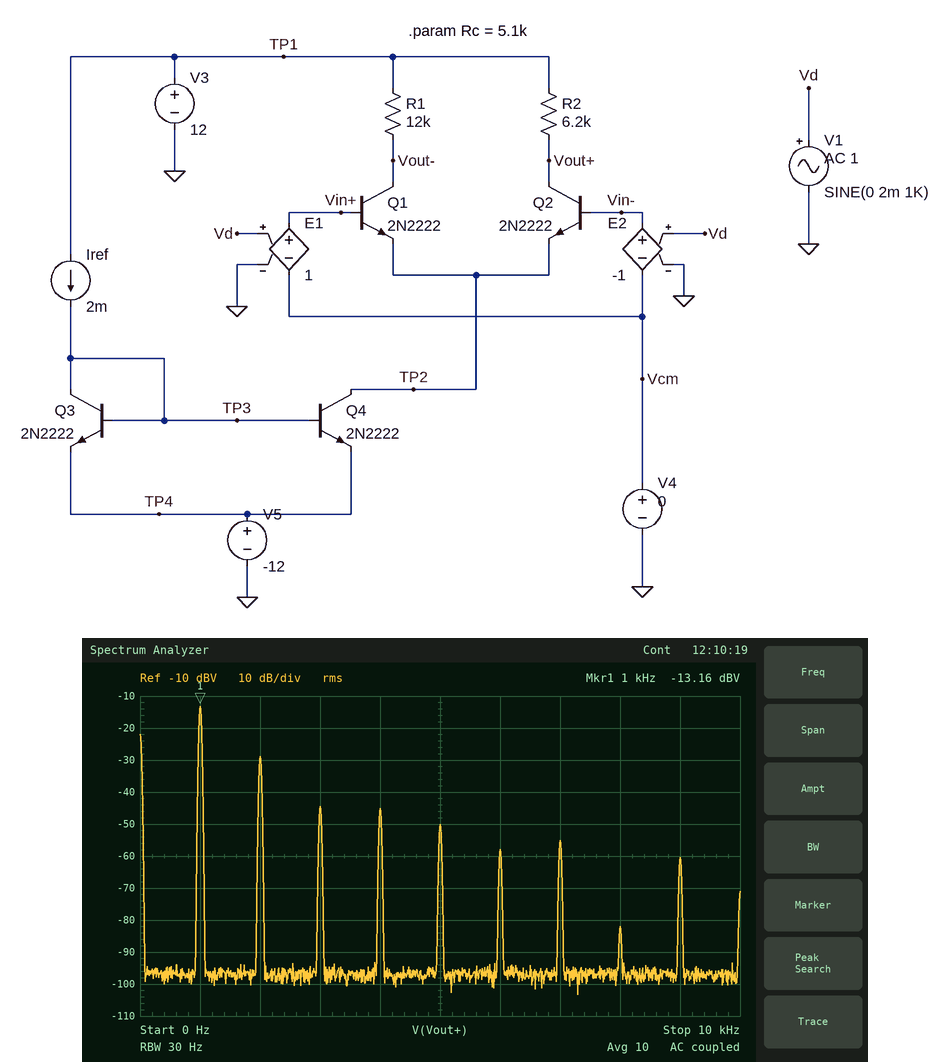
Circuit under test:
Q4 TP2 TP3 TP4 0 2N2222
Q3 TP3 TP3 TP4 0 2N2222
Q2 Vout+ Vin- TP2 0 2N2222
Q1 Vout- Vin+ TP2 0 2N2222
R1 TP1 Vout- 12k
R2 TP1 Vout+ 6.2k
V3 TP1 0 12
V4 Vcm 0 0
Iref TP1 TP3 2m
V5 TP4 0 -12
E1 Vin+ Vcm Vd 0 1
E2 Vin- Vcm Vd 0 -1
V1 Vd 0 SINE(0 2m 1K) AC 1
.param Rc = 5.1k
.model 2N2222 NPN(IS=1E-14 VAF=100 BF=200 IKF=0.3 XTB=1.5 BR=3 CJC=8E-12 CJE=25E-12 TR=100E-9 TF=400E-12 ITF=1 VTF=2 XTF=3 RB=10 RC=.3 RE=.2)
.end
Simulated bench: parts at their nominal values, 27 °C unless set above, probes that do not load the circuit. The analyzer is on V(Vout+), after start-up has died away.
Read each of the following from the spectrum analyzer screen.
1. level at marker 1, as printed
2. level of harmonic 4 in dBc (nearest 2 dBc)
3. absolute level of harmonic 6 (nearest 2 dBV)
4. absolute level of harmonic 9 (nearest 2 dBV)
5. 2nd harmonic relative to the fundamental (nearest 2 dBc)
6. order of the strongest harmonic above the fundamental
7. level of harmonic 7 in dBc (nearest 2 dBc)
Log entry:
-13.16 dBV
-32 dBc
-58 dBV
-60 dBV
-16 dBc
2
-42 dBc
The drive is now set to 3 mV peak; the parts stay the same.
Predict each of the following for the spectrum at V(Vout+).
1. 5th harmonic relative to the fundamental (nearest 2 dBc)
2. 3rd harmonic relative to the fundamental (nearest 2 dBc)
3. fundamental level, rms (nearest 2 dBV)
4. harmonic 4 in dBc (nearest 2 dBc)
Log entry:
-40 dBc
-34 dBc
-10 dBV
-30 dBc
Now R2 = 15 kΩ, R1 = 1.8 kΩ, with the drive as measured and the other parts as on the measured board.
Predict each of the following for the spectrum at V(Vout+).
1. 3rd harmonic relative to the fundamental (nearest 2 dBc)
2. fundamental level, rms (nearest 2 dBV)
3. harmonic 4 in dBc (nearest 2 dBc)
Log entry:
-36 dBc
-42 dBV
-52 dBc
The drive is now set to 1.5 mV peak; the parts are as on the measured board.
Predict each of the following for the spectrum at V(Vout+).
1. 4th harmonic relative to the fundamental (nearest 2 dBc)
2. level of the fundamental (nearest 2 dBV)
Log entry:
-34 dBc
-16 dBV
